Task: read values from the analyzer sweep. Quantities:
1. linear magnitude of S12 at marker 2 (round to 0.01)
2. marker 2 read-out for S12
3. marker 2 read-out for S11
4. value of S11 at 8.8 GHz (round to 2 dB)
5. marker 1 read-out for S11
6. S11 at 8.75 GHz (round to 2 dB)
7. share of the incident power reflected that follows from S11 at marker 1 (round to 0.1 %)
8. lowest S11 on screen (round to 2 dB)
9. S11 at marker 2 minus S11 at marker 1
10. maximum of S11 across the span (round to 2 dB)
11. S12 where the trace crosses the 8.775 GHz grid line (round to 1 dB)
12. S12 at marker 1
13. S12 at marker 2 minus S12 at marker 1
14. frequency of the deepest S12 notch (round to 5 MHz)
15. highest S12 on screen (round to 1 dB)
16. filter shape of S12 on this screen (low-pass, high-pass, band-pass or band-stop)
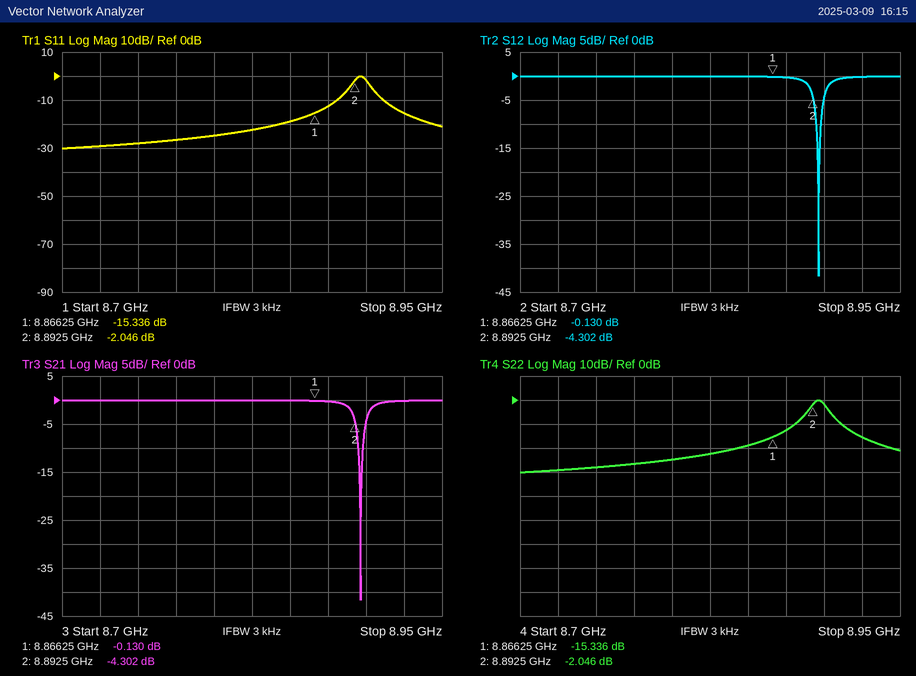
0.61
-4.302 dB
-2.046 dB
-24 dB
-15.336 dB
-28 dB
2.9 %
-30 dB
13.290 dB
0 dB
0 dB
-0.130 dB
-4.172 dB
8.895 GHz
0 dB
band-stop
